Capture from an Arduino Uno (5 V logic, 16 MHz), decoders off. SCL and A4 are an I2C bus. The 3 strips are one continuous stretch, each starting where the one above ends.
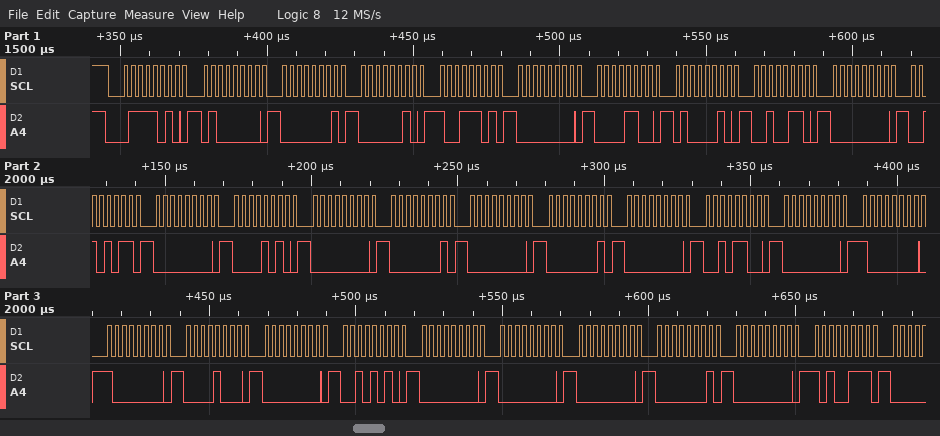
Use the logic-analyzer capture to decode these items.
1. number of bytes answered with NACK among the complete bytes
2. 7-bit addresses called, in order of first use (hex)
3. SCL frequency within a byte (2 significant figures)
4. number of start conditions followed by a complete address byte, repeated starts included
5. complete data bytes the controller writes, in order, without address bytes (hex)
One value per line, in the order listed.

0
0x3D
400 kHz
1
40 01 02 9D 00 0C 42 26 00 2B 00 0A 00 01 00 01 00 2C 00 80 80 08 00 2A 00 00 00 01 00 A7
